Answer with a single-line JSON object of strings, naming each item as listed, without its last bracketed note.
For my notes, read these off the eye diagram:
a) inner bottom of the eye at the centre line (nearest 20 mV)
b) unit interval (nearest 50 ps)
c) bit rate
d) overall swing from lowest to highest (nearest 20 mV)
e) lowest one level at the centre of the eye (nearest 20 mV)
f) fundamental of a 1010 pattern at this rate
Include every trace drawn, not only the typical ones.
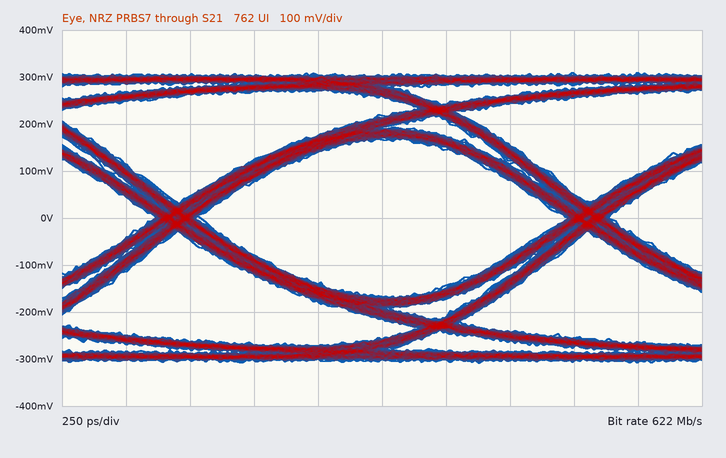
{"inner bottom of the eye at the centre line": "-160 mV", "unit interval": "1.60 ns", "bit rate": "622 Mb/s", "overall swing from lowest to highest": "620 mV", "lowest one level at the centre of the eye": "160 mV", "fundamental of a 1010 pattern at this rate": "311 MHz"}
